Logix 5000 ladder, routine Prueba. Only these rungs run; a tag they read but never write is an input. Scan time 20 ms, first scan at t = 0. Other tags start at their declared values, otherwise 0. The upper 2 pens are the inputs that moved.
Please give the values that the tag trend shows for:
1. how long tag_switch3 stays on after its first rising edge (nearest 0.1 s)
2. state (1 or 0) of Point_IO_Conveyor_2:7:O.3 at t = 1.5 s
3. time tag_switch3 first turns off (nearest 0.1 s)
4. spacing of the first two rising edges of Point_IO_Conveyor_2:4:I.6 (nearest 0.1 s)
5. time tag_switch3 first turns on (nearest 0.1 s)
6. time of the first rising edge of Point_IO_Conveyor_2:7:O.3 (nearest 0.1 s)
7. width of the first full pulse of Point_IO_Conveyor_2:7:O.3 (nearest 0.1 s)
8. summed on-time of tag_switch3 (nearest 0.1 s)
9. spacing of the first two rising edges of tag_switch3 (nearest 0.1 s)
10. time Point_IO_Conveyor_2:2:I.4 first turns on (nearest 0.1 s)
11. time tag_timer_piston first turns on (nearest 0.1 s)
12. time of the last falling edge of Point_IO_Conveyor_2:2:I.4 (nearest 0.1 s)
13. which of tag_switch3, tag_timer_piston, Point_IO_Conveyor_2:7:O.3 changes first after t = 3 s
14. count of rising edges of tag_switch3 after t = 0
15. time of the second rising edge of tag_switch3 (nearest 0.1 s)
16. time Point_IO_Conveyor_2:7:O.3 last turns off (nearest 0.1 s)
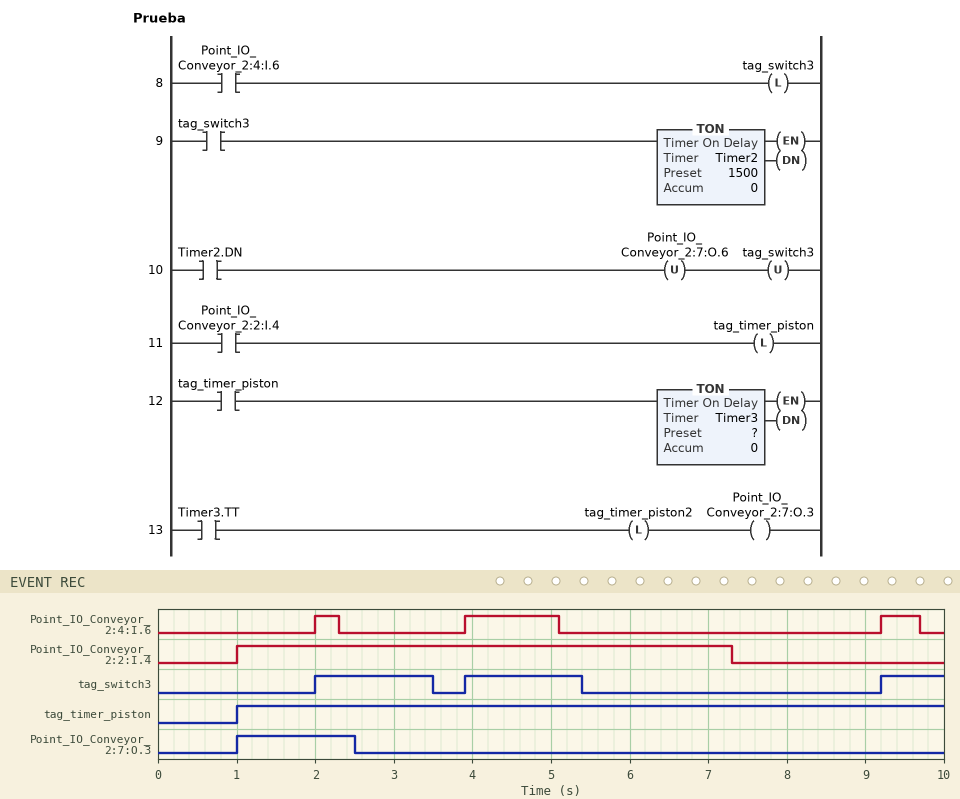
1.5 s
1
3.5 s
1.9 s
2.0 s
1.0 s
1.5 s
3.8 s
1.9 s
1.0 s
1.0 s
7.3 s
tag_switch3
3
3.9 s
2.5 s
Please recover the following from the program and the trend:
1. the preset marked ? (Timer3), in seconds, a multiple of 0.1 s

1.5 s
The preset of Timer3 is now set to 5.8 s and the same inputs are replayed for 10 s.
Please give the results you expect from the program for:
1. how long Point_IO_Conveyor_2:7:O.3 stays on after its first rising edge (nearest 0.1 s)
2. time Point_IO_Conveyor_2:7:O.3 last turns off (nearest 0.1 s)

5.8 s
6.8 s
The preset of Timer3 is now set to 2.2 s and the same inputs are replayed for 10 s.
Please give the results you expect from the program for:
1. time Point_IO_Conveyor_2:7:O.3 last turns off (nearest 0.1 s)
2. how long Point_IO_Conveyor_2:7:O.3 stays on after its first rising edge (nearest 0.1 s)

3.2 s
2.2 s
